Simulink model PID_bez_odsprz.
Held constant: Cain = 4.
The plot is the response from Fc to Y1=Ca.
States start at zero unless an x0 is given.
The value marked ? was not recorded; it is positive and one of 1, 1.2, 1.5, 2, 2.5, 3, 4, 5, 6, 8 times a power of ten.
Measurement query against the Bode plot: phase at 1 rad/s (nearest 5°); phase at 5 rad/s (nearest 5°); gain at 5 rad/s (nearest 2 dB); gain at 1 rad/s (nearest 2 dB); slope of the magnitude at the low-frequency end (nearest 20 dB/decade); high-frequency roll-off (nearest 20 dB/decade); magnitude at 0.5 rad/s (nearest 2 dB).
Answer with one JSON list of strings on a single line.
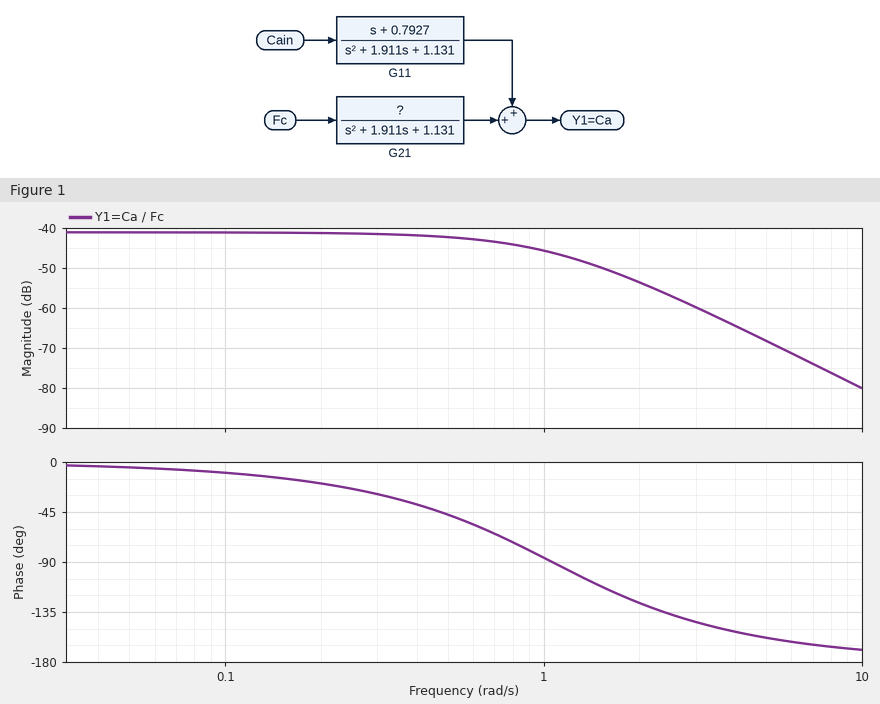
["-85°", "-160°", "-68 dB", "-46 dB", "0 dB/decade", "-40 dB/decade", "-42 dB"]
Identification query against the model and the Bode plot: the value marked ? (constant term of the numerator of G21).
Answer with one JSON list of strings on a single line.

["0.01"]
